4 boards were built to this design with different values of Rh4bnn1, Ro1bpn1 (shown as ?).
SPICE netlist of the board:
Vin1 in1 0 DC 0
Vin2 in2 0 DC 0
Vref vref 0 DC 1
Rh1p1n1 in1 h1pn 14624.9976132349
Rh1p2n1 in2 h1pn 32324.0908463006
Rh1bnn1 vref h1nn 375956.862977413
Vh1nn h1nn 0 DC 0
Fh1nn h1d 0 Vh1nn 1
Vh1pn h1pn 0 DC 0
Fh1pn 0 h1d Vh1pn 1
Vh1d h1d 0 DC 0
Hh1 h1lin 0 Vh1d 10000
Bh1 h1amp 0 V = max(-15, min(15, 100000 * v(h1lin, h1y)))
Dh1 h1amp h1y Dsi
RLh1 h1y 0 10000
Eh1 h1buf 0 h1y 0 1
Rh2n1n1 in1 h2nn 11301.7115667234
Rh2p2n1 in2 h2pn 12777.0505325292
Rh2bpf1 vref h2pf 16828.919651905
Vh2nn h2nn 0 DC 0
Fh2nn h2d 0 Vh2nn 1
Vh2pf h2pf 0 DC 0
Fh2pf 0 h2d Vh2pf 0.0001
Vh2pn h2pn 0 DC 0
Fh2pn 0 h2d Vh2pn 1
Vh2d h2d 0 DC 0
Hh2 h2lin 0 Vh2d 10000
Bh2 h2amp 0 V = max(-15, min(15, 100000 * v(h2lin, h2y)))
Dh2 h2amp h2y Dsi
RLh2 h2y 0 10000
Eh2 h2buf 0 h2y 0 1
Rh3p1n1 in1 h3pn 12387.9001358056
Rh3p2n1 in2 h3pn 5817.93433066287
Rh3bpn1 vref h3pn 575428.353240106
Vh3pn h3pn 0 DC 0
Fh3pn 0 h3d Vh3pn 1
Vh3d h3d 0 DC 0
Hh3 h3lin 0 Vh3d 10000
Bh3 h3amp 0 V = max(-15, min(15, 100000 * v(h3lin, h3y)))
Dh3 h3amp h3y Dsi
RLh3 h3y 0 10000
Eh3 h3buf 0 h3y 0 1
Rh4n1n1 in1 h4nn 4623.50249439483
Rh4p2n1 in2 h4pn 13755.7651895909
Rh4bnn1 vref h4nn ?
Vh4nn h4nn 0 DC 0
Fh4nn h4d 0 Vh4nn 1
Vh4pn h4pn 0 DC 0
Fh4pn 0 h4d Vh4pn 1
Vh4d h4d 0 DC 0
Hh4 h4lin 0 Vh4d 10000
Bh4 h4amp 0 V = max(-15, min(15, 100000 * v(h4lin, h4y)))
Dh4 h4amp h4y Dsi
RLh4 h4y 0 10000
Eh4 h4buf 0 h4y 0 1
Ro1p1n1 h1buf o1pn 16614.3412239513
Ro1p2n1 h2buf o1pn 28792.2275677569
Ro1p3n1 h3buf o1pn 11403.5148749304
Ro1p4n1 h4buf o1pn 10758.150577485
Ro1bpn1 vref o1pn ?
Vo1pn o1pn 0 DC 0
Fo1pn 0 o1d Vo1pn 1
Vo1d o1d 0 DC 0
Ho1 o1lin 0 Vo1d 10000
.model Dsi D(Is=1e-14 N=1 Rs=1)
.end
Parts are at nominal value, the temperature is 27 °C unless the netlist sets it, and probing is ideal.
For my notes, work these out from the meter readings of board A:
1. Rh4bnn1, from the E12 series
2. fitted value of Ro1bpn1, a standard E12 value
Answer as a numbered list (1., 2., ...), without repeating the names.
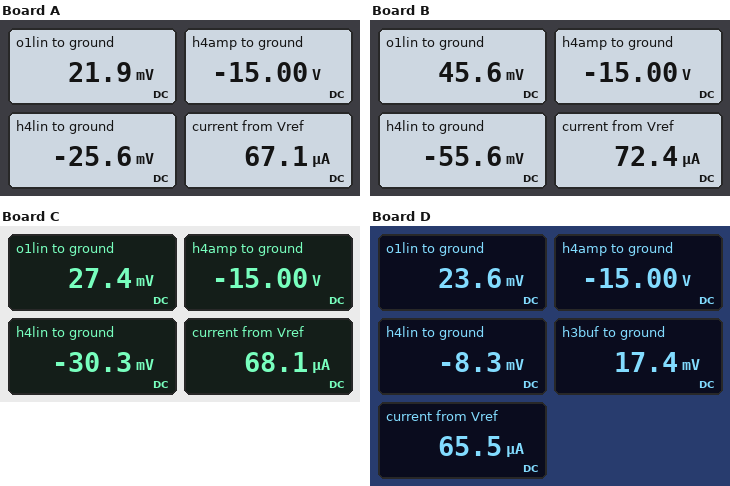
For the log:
1. 390 kΩ
2. 1.5 MΩ
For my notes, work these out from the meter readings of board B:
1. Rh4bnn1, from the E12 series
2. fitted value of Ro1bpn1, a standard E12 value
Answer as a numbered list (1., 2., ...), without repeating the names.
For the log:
1. 180 kΩ
2. 330 kΩ
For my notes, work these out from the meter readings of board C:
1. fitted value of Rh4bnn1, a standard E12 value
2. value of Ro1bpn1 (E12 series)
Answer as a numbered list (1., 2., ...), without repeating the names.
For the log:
1. 330 kΩ
2. 820 kΩ
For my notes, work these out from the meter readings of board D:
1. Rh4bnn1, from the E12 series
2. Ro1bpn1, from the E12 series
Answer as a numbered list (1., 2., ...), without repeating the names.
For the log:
1. 1.2 MΩ
2. 1.2 MΩ
